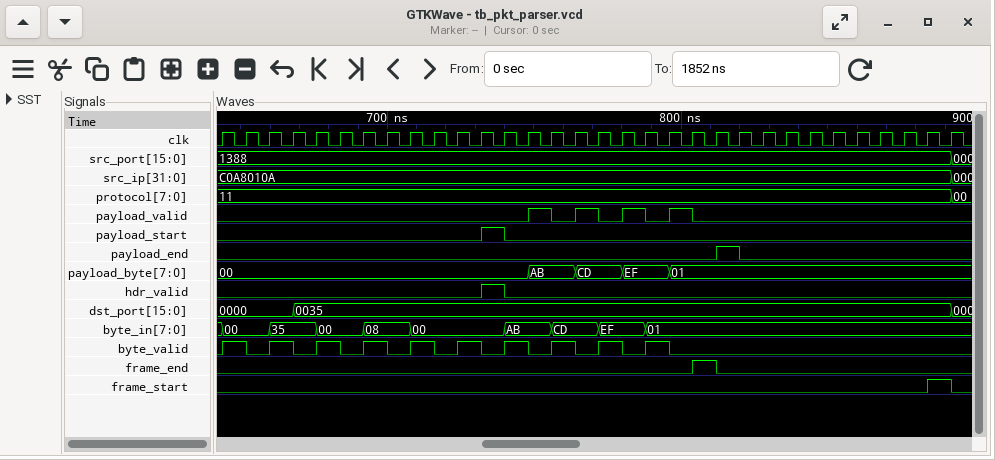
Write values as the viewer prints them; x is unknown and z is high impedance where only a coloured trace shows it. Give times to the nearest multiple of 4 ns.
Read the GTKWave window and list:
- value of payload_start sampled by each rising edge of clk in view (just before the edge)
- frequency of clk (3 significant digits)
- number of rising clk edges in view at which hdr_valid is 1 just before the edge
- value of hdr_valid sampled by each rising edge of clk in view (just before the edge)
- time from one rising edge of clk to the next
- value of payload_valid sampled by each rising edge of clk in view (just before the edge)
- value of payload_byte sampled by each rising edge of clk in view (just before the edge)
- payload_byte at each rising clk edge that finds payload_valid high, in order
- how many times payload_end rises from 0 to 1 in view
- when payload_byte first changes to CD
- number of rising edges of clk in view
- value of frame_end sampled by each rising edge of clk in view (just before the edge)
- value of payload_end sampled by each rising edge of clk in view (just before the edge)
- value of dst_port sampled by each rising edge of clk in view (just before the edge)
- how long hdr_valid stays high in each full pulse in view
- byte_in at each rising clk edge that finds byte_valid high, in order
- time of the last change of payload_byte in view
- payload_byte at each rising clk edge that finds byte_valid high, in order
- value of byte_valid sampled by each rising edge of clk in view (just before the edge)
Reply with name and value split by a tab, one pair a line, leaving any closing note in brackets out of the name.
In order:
value of payload_start sampled by each rising edge of clk in view	0 0 0 0 0 0 0 0 0 0 0 0 1 0 0 0 0 0 0 0 0 0 0 0 0 0 0 0 0 0 0 0
frequency of clk	125 MHz
number of rising clk edges in view at which hdr_valid is 1 just before the edge	1
value of hdr_valid sampled by each rising edge of clk in view	0 0 0 0 0 0 0 0 0 0 0 0 1 0 0 0 0 0 0 0 0 0 0 0 0 0 0 0 0 0 0 0
time from one rising edge of clk to the next	8 ns
value of payload_valid sampled by each rising edge of clk in view	0 0 0 0 0 0 0 0 0 0 0 0 0 0 1 0 1 0 1 0 1 0 0 0 0 0 0 0 0 0 0 0
value of payload_byte sampled by each rising edge of clk in view	00, 00, 00, 00, 00, 00, 00, 00, 00, 00, 00, 00, 00, 00, AB, AB, CD, CD, EF, EF, 01, 01, 01, 01, 01, 01, 01, 01, 01, 01, 01, 01
payload_byte at each rising clk edge that finds payload_valid high, in order	AB, CD, EF, 01
how many times payload_end rises from 0 to 1 in view	1
when payload_byte first changes to CD	764 ns
number of rising edges of clk in view	32
value of frame_end sampled by each rising edge of clk in view	0 0 0 0 0 0 0 0 0 0 0 0 0 0 0 0 0 0 0 0 0 1 0 0 0 0 0 0 0 0 0 0
value of payload_end sampled by each rising edge of clk in view	0 0 0 0 0 0 0 0 0 0 0 0 0 0 0 0 0 0 0 0 0 0 1 0 0 0 0 0 0 0 0 0
value of dst_port sampled by each rising edge of clk in view	0000, 0000, 0000, 0000, 0035, 0035, 0035, 0035, 0035, 0035, 0035, 0035, 0035, 0035, 0035, 0035, 0035, 0035, 0035, 0035, 0035, 0035, 0035, 0035, 0035, 0035, 0035, 0035, 0035, 0035, 0035, 0035
how long hdr_valid stays high in each full pulse in view	8 ns
byte_in at each rising clk edge that finds byte_valid high, in order	00, 35, 00, 08, 00, 00, AB, CD, EF, 01
time of the last change of payload_byte in view	796 ns
payload_byte at each rising clk edge that finds byte_valid high, in order	00, 00, 00, 00, 00, 00, 00, AB, CD, EF
value of byte_valid sampled by each rising edge of clk in view	0 1 0 1 0 1 0 1 0 1 0 1 0 1 0 1 0 1 0 1 0 0 0 0 0 0 0 0 0 0 0 0
